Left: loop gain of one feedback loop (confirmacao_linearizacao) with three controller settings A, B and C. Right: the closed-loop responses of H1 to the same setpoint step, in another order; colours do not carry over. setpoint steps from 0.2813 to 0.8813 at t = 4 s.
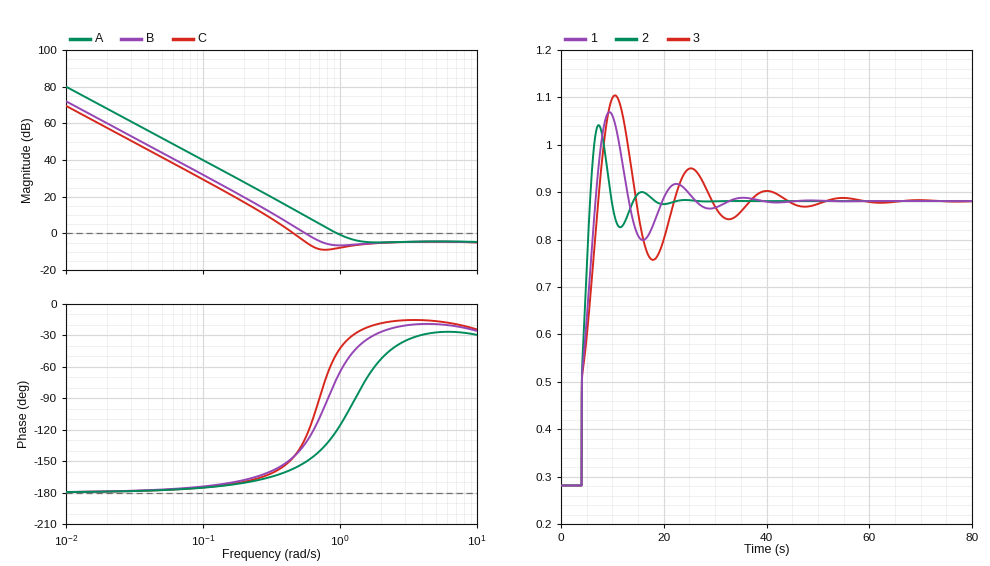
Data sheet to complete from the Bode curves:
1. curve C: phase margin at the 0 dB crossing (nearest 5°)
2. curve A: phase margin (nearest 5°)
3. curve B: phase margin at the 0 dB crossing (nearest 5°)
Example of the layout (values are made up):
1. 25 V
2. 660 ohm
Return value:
1. 35°
2. 60°
3. 45°
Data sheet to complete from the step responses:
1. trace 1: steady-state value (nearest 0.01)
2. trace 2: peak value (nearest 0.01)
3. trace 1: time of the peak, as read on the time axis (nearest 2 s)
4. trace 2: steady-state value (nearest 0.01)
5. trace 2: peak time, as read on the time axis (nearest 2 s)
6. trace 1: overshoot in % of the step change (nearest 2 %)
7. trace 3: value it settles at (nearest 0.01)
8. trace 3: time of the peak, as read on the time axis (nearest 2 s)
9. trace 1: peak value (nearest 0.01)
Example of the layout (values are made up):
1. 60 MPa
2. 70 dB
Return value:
1. 0.88
2. 1.04
3. 10 s
4. 0.88
5. 8 s
6. 32 %
7. 0.88
8. 10 s
9. 1.07
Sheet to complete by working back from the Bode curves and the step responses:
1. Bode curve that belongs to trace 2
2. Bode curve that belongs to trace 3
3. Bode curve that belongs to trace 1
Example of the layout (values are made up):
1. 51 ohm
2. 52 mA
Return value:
1. A
2. C
3. B
